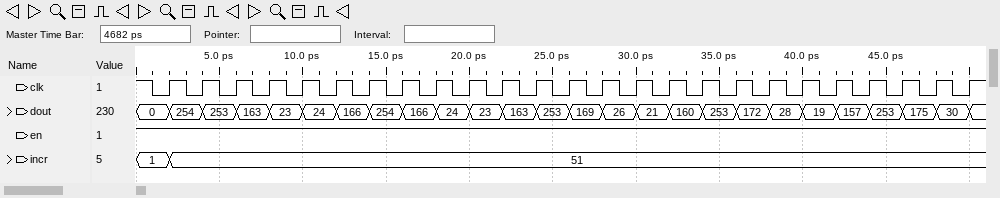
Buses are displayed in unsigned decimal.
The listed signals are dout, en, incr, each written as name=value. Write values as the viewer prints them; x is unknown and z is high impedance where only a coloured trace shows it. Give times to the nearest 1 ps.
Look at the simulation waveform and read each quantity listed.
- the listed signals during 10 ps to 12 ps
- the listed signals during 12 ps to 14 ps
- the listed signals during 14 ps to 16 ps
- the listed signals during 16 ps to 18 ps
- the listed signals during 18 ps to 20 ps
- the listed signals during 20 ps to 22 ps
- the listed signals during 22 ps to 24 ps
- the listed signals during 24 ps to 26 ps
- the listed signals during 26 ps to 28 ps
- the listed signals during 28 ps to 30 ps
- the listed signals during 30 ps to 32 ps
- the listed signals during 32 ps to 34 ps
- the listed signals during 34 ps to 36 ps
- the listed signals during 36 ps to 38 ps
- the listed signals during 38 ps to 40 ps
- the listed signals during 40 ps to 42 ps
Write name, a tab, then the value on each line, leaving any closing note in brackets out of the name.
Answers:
the listed signals during 10 ps to 12 ps	dout=24, en=1, incr=51
the listed signals during 12 ps to 14 ps	dout=166, en=1, incr=51
the listed signals during 14 ps to 16 ps	dout=254, en=1, incr=51
the listed signals during 16 ps to 18 ps	dout=166, en=1, incr=51
the listed signals during 18 ps to 20 ps	dout=24, en=1, incr=51
the listed signals during 20 ps to 22 ps	dout=23, en=1, incr=51
the listed signals during 22 ps to 24 ps	dout=163, en=1, incr=51
the listed signals during 24 ps to 26 ps	dout=253, en=1, incr=51
the listed signals during 26 ps to 28 ps	dout=169, en=1, incr=51
the listed signals during 28 ps to 30 ps	dout=26, en=1, incr=51
the listed signals during 30 ps to 32 ps	dout=21, en=1, incr=51
the listed signals during 32 ps to 34 ps	dout=160, en=1, incr=51
the listed signals during 34 ps to 36 ps	dout=253, en=1, incr=51
the listed signals during 36 ps to 38 ps	dout=172, en=1, incr=51
the listed signals during 38 ps to 40 ps	dout=28, en=1, incr=51
the listed signals during 40 ps to 42 ps	dout=19, en=1, incr=51
